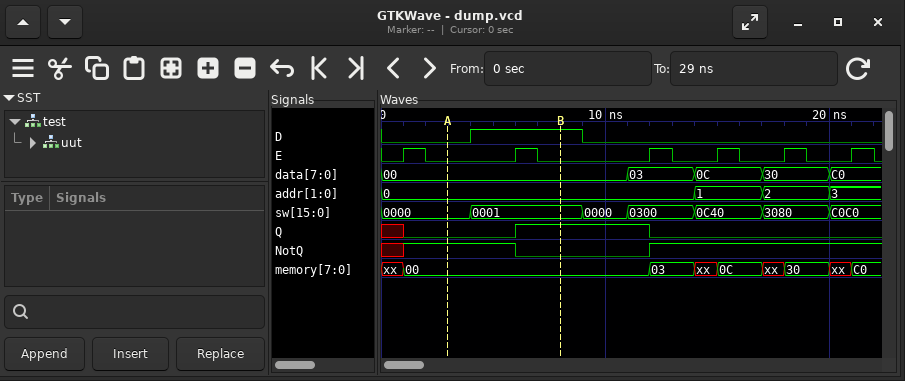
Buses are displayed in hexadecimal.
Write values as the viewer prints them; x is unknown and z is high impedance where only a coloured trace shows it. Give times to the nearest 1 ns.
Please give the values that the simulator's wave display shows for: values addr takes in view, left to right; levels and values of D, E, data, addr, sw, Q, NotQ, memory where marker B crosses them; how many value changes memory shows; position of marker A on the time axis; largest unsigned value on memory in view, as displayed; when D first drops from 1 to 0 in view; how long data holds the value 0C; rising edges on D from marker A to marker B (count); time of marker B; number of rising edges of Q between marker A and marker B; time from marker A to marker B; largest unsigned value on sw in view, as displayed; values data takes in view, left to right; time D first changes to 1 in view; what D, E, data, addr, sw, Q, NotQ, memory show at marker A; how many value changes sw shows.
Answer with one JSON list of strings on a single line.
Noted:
["0, 1, 2, 3", "D=1, E=0, data=00, addr=0, sw=0001, Q=1, NotQ=0, memory=00", "8", "3 ns", "C0", "9 ns", "3 ns", "1", "8 ns", "1", "5 ns", "C0C0", "00, 03, 0C, 30, C0", "4 ns", "D=0, E=0, data=00, addr=0, sw=0000, Q=0, NotQ=1, memory=00", "6"]
